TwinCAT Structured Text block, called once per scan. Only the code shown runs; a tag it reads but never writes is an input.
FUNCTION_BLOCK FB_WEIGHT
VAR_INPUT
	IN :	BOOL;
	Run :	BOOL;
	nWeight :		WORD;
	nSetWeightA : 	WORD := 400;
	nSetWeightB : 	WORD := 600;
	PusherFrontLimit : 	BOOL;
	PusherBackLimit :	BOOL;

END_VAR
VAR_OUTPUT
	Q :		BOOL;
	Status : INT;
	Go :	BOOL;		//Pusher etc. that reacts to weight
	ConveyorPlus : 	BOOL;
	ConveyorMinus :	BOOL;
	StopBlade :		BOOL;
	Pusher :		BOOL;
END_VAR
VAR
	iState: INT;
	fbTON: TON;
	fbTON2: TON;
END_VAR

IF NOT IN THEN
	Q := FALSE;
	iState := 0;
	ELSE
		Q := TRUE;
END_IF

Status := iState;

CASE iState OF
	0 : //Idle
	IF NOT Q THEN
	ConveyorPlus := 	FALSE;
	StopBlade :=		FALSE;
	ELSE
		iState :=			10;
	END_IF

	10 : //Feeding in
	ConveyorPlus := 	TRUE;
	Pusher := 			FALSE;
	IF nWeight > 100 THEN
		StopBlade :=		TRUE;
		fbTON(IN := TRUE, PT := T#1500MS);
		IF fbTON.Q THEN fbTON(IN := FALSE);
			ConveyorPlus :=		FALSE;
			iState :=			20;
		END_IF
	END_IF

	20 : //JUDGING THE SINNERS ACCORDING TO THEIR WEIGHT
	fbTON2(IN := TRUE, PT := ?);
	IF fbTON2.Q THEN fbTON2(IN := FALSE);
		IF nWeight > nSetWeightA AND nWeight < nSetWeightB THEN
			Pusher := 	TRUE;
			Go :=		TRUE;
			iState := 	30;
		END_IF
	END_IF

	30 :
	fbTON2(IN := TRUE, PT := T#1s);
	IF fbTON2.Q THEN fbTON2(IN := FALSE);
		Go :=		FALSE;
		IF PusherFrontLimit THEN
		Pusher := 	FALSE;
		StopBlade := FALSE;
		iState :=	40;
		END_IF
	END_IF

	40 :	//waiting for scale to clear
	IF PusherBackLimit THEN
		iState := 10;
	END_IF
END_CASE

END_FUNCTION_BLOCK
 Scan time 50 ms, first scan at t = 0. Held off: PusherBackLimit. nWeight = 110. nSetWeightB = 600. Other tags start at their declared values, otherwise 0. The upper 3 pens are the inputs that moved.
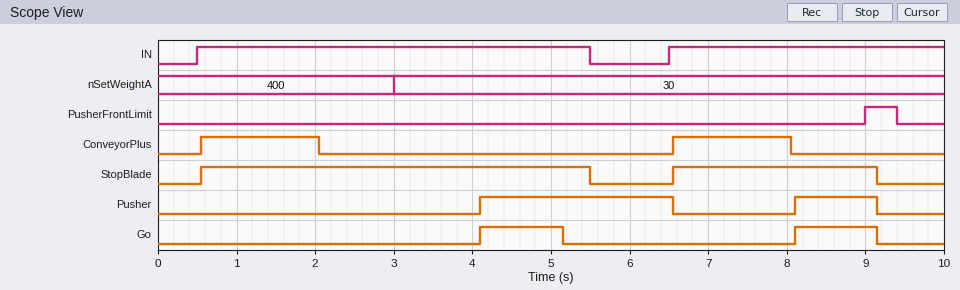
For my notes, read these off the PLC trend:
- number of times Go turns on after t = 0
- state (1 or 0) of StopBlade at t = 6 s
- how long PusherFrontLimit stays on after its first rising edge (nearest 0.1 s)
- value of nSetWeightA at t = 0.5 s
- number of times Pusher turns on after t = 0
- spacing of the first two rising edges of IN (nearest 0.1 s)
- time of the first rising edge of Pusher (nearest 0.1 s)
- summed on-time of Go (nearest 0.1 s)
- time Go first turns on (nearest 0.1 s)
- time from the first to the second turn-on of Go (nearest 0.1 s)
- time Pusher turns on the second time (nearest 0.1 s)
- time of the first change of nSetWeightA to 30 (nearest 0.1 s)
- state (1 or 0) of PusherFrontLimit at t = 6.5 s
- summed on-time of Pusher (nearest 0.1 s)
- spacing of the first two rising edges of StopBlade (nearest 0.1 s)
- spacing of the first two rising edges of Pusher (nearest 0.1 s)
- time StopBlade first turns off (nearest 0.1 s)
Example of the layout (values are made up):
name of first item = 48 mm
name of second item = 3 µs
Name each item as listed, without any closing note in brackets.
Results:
number of times Go turns on after t = 0 = 2
state (1 or 0) of StopBlade at t = 6 s = 0
how long PusherFrontLimit stays on after its first rising edge = 0.4 s
value of nSetWeightA at t = 0.5 s = 400
number of times Pusher turns on after t = 0 = 2
spacing of the first two rising edges of IN = 6.0 s
time of the first rising edge of Pusher = 4.1 s
summed on-time of Go = 2.1 s
time Go first turns on = 4.1 s
time from the first to the second turn-on of Go = 4.0 s
time Pusher turns on the second time = 8.1 s
time of the first change of nSetWeightA to 30 = 3.0 s
state (1 or 0) of PusherFrontLimit at t = 6.5 s = 0
summed on-time of Pusher = 3.5 s
spacing of the first two rising edges of StopBlade = 6.0 s
spacing of the first two rising edges of Pusher = 4.0 s
time StopBlade first turns off = 5.5 s
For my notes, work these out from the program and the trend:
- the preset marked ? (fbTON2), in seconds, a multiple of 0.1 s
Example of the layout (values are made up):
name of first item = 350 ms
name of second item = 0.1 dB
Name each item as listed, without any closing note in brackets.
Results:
the preset marked ? (fbTON2), in seconds, a multiple of 0.1 s = 2.0 s
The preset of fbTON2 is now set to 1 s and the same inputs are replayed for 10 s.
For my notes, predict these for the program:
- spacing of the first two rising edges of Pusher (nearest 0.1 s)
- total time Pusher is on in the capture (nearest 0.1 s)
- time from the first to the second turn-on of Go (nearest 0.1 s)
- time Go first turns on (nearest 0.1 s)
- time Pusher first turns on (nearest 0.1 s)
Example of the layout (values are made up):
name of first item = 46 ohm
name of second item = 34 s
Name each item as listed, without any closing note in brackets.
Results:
spacing of the first two rising edges of Pusher = 5.0 s
total time Pusher is on in the capture = 4.5 s
time from the first to the second turn-on of Go = 5.0 s
time Go first turns on = 3.1 s
time Pusher first turns on = 3.1 s
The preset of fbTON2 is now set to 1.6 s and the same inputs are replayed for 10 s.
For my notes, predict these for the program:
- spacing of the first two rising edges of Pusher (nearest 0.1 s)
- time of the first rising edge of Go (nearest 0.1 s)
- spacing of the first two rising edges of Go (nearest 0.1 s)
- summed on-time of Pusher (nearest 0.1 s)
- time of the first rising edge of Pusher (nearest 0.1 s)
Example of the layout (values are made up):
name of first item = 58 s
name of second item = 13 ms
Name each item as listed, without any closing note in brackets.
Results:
spacing of the first two rising edges of Pusher = 4.4 s
time of the first rising edge of Go = 3.7 s
spacing of the first two rising edges of Go = 4.4 s
summed on-time of Pusher = 3.9 s
time of the first rising edge of Pusher = 3.7 s
